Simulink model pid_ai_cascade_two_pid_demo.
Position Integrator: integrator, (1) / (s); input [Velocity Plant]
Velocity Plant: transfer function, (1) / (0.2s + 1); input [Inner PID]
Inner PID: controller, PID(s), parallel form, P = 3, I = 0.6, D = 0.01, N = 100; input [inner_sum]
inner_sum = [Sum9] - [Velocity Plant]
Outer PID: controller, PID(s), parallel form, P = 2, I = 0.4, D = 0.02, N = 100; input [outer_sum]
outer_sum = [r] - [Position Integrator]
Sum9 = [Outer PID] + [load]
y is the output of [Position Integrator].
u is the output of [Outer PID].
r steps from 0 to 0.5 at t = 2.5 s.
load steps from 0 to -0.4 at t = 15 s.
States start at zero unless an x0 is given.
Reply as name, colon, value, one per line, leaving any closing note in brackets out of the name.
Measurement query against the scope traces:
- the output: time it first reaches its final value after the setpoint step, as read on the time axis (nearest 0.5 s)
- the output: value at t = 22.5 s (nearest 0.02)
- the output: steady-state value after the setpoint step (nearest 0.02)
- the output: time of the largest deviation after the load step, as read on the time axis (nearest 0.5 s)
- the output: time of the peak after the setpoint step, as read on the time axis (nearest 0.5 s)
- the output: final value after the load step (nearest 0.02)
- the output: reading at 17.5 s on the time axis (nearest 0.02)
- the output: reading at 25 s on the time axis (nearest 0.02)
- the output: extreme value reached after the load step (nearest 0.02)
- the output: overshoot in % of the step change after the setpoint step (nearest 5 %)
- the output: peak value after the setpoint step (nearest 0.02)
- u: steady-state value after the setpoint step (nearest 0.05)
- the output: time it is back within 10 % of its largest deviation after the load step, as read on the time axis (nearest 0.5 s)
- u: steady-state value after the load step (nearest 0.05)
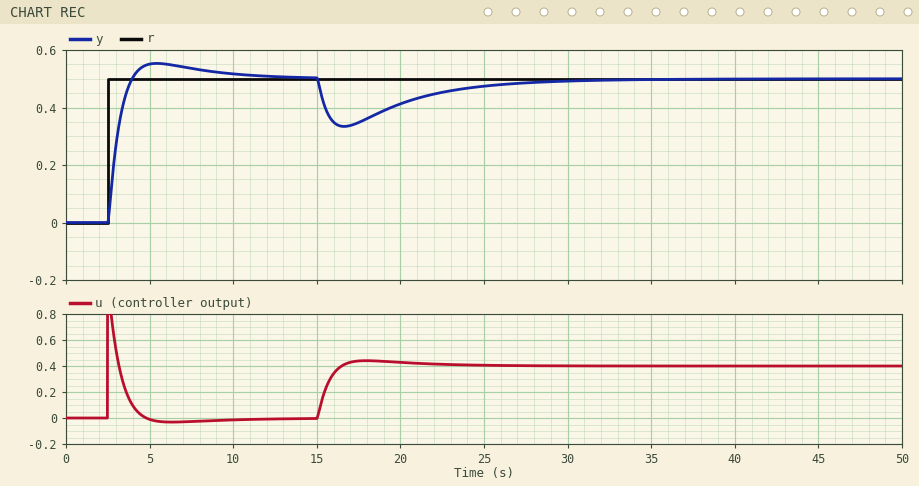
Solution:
the output: time it first reaches its final value after the setpoint step, as read on the time axis: 4.0 s
the output: value at t = 22.5 s: 0.46
the output: steady-state value after the setpoint step: 0.50
the output: time of the largest deviation after the load step, as read on the time axis: 16.5 s
the output: time of the peak after the setpoint step, as read on the time axis: 5.5 s
the output: final value after the load step: 0.50
the output: reading at 17.5 s on the time axis: 0.34
the output: reading at 25 s on the time axis: 0.48
the output: extreme value reached after the load step: 0.34
the output: overshoot in % of the step change after the setpoint step: 10 %
the output: peak value after the setpoint step: 0.56
u: steady-state value after the setpoint step: 0.00
the output: time it is back within 10 % of its largest deviation after the load step, as read on the time axis: 27.0 s
u: steady-state value after the load step: 0.40
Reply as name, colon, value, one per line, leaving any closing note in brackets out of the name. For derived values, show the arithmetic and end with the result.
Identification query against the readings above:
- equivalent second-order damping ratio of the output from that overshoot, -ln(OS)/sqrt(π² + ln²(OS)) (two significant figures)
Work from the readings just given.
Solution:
equivalent second-order damping ratio of the output from that overshoot, -ln(OS)/sqrt(π² + ln²(OS)): ln(0.1) = -2.303; 2.303 / sqrt(9.870 + 5.302) = 0.59
